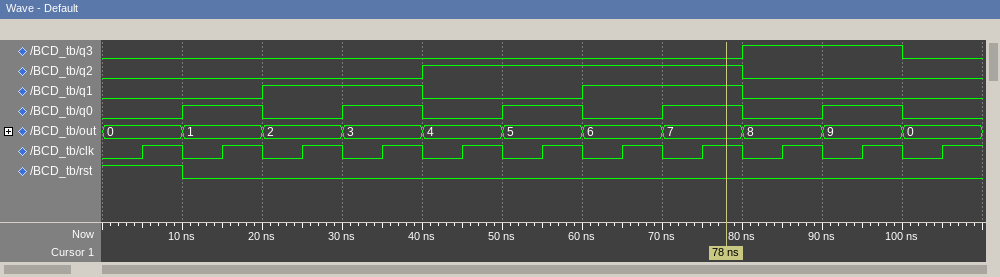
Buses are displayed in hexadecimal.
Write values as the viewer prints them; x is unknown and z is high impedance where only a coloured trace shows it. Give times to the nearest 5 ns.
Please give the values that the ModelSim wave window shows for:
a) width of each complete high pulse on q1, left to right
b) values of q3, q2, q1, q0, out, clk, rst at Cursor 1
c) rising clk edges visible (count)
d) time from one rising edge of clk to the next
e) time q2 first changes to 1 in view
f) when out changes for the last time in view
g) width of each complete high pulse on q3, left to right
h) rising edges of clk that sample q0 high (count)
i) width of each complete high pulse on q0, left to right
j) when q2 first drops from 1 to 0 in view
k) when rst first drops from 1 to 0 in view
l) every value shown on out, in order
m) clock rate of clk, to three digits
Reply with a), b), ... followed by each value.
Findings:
a) 20 ns, 20 ns
b) q3=0, q2=1, q1=1, q0=1, out=7, clk=1, rst=0
c) 11
d) 10 ns
e) 40 ns
f) 100 ns
g) 20 ns
h) 5
i) 10 ns, 10 ns, 10 ns, 10 ns, 10 ns
j) 80 ns
k) 10 ns
l) 0, 1, 2, 3, 4, 5, 6, 7, 8, 9, 0
m) 100 MHz
